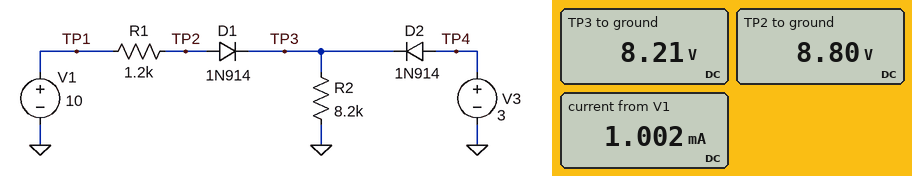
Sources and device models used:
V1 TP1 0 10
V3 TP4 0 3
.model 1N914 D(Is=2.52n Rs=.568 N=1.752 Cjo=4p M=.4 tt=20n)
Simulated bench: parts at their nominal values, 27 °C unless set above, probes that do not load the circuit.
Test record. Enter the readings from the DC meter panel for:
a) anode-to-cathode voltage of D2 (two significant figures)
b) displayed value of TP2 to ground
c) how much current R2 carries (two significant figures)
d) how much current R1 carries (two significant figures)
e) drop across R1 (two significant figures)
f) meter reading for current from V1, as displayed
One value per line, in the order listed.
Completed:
-5.2 V
8.80 V
1.0 mA
1.0 mA
1.2 V
1.002 mA
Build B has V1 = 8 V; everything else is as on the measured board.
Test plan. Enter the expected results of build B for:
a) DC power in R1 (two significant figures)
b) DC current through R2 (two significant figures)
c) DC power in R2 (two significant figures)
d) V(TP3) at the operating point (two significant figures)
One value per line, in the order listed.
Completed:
750 µW
790 µA
5.1 mW
6.5 V
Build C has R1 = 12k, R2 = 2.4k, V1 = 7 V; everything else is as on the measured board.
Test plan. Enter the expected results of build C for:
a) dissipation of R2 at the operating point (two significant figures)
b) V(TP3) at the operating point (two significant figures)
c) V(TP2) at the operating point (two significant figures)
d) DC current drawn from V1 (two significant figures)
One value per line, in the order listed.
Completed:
2.5 mW
2.4 V
3.0 V
340 µA
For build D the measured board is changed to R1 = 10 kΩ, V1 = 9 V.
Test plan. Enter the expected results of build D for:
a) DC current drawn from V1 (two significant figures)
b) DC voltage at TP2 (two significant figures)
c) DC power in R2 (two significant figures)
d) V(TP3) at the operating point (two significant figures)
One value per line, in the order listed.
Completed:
460 µA
4.4 V
1.8 mW
3.8 V
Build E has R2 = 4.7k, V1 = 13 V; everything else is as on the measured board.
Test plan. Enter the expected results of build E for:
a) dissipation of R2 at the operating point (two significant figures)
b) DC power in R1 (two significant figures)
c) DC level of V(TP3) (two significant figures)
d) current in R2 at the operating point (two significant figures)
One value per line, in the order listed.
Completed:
21 mW
5.3 mW
9.9 V
2.1 mA
